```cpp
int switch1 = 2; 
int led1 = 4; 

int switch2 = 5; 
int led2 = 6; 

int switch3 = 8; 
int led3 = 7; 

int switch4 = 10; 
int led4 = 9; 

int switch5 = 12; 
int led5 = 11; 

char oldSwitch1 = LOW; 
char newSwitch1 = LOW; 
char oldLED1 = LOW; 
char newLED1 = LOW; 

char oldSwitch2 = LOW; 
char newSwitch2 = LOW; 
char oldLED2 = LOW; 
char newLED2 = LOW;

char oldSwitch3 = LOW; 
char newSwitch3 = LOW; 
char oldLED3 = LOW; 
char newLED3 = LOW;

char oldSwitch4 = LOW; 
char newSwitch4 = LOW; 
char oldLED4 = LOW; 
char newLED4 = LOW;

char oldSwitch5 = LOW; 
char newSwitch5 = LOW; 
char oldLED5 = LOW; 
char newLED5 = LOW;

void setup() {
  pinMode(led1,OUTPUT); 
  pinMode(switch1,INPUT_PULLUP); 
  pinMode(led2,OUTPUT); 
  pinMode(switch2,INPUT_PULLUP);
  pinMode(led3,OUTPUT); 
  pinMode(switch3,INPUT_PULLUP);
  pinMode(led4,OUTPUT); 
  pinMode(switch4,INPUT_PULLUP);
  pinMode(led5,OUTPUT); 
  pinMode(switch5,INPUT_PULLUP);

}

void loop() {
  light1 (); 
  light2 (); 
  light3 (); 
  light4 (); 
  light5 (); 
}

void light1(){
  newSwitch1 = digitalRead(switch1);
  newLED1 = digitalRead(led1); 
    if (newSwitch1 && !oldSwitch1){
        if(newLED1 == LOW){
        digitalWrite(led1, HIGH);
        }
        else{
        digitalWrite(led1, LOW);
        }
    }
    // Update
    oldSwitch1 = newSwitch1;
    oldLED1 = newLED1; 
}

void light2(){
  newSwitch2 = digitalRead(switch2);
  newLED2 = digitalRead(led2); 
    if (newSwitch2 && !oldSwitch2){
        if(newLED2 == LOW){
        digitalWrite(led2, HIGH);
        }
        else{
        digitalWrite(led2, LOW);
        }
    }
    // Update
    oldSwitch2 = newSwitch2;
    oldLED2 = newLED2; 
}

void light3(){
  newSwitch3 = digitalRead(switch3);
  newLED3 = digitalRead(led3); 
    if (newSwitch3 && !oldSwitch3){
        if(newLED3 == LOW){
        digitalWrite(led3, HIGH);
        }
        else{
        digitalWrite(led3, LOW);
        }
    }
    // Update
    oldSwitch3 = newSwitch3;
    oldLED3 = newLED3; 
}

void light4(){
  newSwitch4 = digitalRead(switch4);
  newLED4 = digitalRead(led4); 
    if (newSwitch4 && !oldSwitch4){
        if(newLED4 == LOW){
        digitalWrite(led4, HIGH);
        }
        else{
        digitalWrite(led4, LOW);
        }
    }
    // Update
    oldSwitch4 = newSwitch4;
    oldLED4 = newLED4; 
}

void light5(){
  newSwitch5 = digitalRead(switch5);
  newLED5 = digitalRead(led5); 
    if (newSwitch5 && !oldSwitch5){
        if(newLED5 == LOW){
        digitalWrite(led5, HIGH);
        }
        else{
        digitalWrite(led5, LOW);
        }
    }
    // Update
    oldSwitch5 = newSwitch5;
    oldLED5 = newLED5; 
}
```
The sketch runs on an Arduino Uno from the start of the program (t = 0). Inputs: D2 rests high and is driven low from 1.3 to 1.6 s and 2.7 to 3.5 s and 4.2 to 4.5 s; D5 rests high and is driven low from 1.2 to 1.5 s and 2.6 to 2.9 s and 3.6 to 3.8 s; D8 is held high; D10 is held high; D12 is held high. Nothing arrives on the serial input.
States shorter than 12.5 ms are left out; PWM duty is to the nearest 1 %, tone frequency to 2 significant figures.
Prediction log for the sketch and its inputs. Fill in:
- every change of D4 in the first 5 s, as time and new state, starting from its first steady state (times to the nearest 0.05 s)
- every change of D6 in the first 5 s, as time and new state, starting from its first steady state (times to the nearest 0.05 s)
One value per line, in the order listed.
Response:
0 s high; 1.6 s low; 3.5 s high; 4.5 s low
0 s high; 1.5 s low; 2.9 s high; 3.8 s low
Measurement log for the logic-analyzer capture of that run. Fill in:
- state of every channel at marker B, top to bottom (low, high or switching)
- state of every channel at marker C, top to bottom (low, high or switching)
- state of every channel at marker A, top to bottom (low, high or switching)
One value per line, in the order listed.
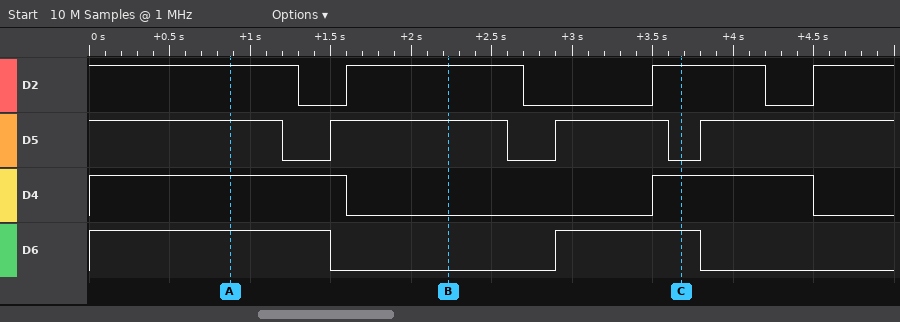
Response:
D2 high, D5 high, D4 low, D6 low
D2 high, D5 low, D4 high, D6 high
D2 high, D5 high, D4 high, D6 high
